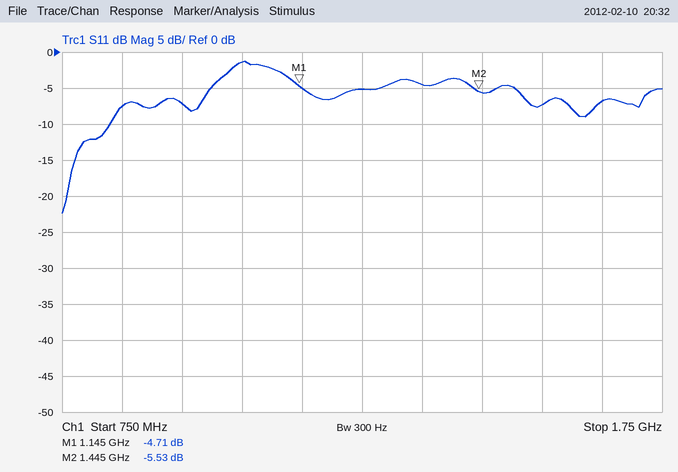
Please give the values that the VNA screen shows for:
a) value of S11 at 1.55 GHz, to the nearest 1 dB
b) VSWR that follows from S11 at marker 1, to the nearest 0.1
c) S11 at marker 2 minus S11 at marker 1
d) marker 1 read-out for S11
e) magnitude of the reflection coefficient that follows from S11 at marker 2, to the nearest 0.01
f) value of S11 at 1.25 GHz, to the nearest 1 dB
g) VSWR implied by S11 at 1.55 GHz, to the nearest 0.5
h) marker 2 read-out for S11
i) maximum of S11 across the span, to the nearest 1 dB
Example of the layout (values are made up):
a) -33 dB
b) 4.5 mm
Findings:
a) -7 dB
b) 3.8
c) -0.82 dB
d) -4.71 dB
e) 0.53
f) -5 dB
g) 2.5
h) -5.53 dB
i) -1 dB
